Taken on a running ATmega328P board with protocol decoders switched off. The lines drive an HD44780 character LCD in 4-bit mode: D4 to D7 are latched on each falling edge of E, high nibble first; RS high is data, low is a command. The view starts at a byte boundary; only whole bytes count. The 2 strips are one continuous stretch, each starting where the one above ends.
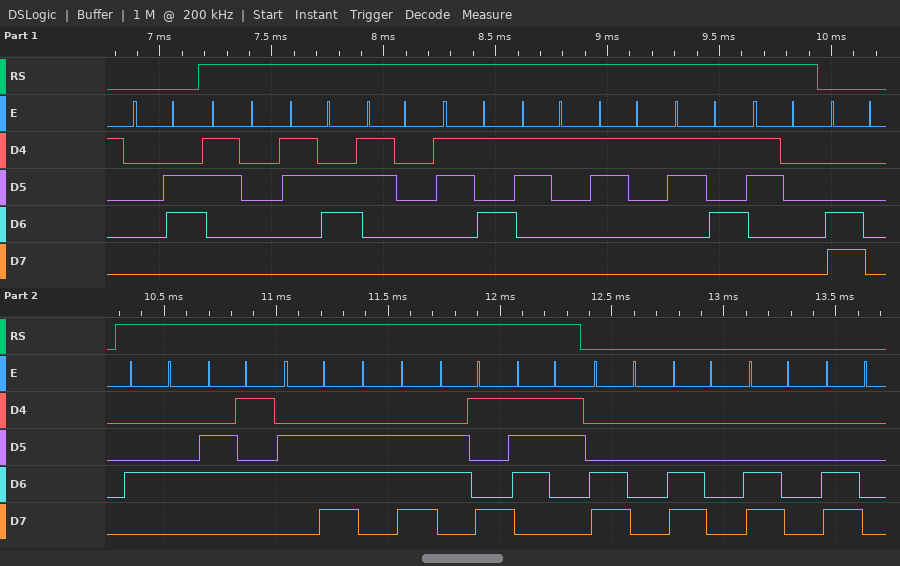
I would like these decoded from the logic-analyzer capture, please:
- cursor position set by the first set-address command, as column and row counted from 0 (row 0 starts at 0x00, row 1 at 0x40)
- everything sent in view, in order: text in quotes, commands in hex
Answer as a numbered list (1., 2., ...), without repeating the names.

1. column 0, row 1
2. 0x06 "06051150" 0xC0 "Dennis" 0xC0 0xC0 0xC0 0xC0
